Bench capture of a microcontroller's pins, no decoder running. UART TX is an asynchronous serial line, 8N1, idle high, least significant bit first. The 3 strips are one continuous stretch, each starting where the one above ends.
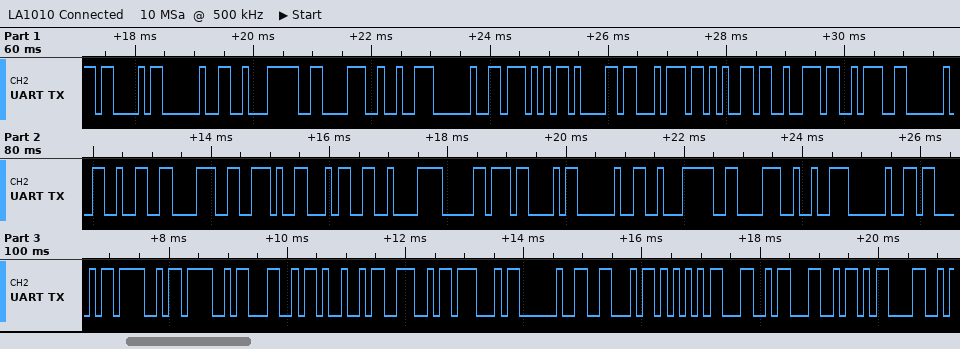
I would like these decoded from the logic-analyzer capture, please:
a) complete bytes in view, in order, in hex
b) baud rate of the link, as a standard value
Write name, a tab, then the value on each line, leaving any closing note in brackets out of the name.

complete bytes in view, in order, in hex	43 20 E2 86 92 20 57 61 74 65 72 3A 20 32 38 2E 34 C2 B0 43 20 E2 86 92 20 43 4F 4F 4C 49 4E 47 20 46 55 4C 4C 0D
baud rate of the link, as a standard value	9600 baud
